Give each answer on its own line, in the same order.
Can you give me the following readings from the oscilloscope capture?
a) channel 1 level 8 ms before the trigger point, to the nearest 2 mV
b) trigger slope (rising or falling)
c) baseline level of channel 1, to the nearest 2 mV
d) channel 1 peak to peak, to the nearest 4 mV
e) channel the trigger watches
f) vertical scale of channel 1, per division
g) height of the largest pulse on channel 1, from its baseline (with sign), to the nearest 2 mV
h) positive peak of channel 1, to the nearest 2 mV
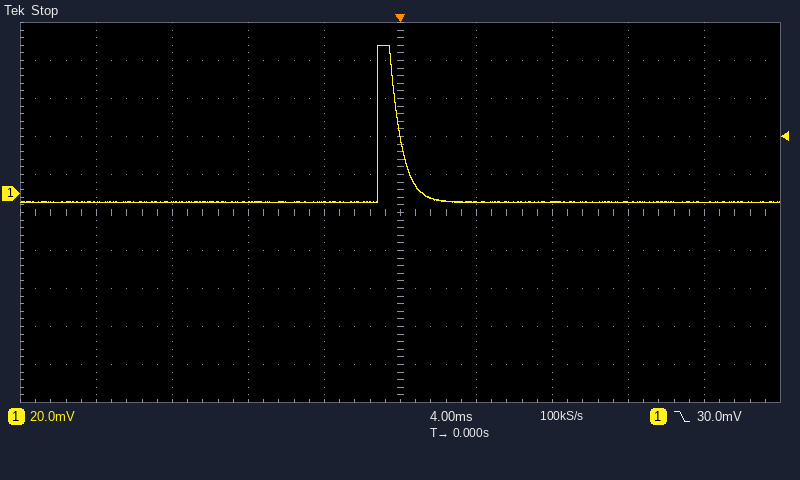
-4 mV
falling
-4 mV
84 mV
channel 1
20 mV
+82 mV
78 mV
